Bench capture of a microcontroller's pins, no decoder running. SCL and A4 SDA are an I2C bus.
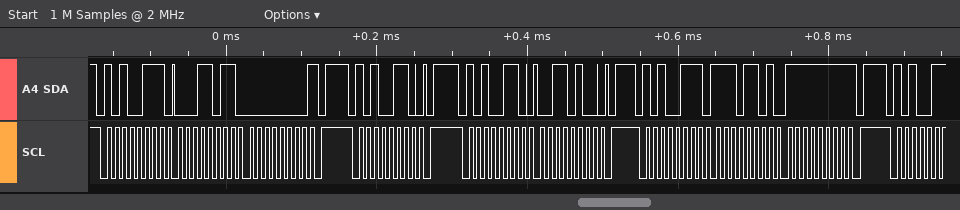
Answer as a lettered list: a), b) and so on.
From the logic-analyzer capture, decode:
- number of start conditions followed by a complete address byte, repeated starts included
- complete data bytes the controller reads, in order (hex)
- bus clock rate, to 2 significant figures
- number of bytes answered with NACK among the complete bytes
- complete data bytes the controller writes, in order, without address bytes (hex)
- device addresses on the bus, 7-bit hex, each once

a) 4
b) 1B 00 ED FF
c) 100 kHz
d) 2
e) 34
f) 0x53
